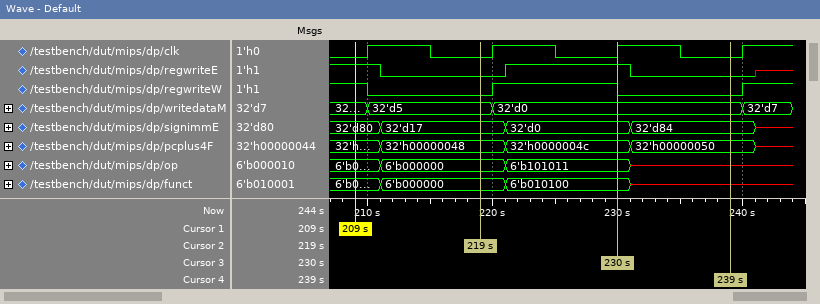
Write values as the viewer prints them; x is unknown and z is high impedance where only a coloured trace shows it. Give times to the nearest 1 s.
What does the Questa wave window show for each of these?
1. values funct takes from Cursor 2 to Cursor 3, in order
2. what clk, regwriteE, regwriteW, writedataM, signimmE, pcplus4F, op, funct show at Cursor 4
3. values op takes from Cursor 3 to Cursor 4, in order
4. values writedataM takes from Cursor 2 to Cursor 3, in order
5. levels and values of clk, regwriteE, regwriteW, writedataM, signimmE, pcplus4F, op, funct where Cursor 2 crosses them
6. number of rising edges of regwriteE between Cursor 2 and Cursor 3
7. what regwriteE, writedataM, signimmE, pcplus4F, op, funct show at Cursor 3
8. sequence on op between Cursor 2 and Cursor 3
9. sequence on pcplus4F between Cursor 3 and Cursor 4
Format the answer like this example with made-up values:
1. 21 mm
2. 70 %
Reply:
1. 6'b000000, 6'b010100
2. clk=0, regwriteE=0, regwriteW=0, writedataM=32'd0, signimmE=32'd84, pcplus4F=32'h00000050, op=x, funct=x
3. 6'b101011, x
4. 32'd5, 32'd0
5. clk=0, regwriteE=0, regwriteW=0, writedataM=32'd5, signimmE=32'd17, pcplus4F=32'h00000048, op=6'b000000, funct=6'b000000
6. 1
7. regwriteE=1, writedataM=32'd0, signimmE=32'd0, pcplus4F=32'h0000004c, op=6'b101011, funct=6'b010100
8. 6'b000000, 6'b101011
9. 32'h0000004c, 32'h00000050
